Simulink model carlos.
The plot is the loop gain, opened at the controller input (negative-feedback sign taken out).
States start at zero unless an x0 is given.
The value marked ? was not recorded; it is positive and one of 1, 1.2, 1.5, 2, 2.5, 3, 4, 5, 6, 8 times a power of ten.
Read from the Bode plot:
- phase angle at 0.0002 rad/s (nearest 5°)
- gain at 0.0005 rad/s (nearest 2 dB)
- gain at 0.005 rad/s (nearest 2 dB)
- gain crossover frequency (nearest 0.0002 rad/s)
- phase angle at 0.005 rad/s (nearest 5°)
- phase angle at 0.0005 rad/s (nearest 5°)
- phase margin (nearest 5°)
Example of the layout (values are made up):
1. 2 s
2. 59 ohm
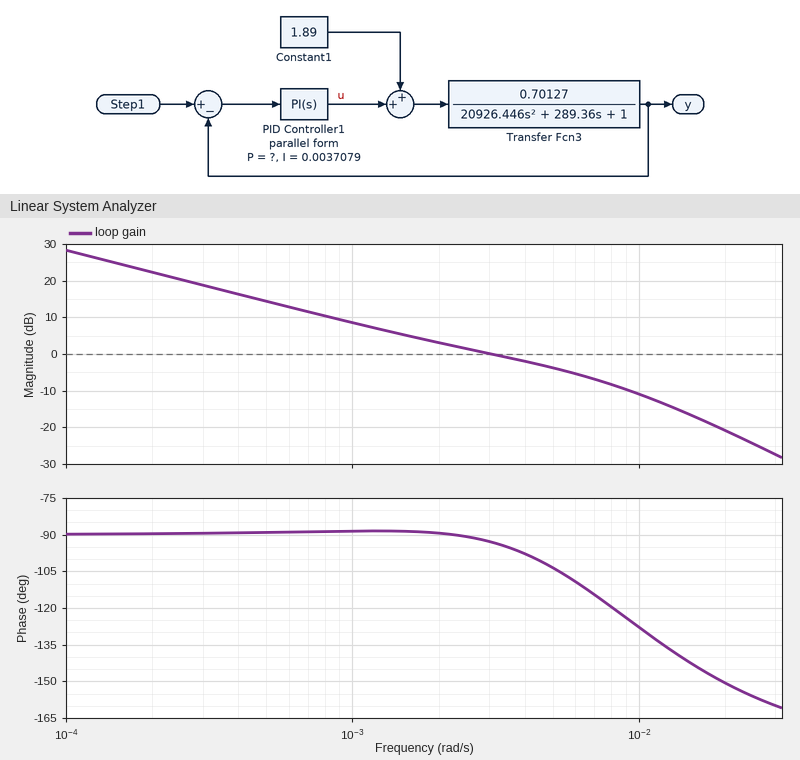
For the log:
1. -90°
2. 14 dB
3. -4 dB
4. 0.0030 rad/s
5. -105°
6. -90°
7. 85°
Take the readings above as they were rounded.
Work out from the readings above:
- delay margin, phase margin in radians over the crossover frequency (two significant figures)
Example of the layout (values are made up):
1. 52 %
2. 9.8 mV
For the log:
1. 490 s
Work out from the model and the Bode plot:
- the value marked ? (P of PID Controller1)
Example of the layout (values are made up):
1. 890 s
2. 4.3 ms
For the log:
1. 1.2
